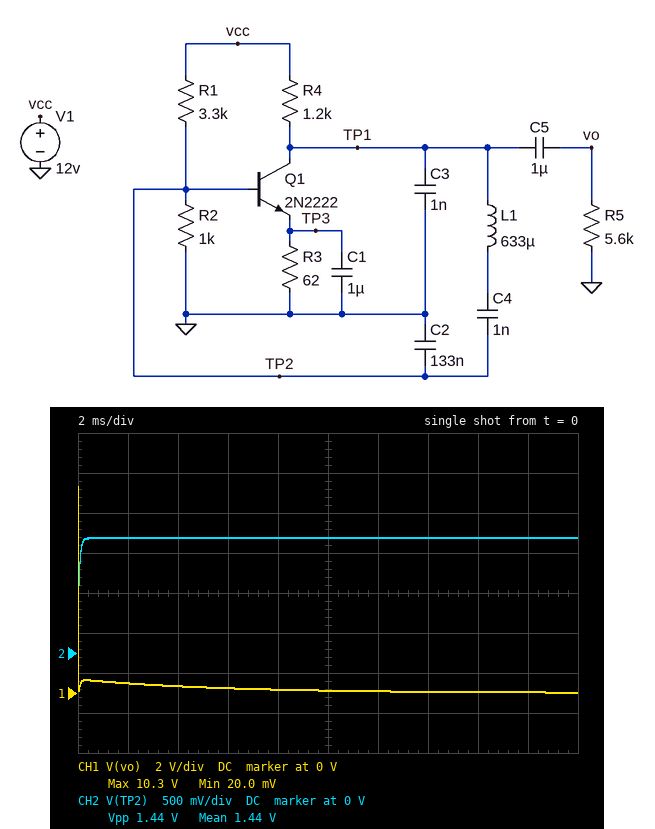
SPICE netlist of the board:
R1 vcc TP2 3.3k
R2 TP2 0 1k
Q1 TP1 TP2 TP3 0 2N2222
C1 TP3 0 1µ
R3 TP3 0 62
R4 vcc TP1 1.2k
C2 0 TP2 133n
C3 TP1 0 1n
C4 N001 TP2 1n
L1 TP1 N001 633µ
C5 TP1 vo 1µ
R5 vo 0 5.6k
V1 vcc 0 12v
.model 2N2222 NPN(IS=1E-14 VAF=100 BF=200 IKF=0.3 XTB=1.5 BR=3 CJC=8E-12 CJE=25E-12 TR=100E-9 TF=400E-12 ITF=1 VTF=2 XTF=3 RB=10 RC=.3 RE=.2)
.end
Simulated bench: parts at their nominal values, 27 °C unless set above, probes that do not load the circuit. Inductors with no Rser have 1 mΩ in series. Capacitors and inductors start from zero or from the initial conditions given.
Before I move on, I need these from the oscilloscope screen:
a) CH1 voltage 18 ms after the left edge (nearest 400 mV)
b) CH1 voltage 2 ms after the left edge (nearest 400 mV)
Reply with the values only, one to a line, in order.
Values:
0 V
400 mV
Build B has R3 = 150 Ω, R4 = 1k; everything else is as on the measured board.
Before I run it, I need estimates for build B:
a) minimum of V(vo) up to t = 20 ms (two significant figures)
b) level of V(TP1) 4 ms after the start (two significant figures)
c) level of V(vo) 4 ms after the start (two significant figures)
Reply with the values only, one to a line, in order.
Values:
50 mV
1.7 V
820 mV
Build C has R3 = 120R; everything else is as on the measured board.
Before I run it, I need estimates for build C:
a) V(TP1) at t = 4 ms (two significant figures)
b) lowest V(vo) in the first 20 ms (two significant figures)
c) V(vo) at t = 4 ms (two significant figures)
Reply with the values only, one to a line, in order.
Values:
1.2 V
36 mV
600 mV
